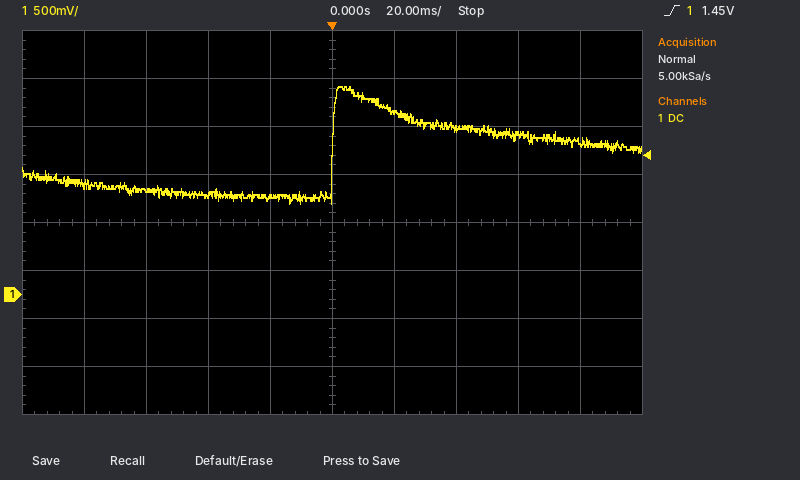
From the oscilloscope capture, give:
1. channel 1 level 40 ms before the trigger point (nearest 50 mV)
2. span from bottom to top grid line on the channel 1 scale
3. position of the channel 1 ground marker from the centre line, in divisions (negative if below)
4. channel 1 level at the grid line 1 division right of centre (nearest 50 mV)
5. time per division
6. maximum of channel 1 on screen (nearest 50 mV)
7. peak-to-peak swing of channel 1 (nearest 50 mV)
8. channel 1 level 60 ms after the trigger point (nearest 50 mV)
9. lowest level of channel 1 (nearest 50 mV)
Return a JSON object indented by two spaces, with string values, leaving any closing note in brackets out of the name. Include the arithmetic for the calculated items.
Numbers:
{
  "channel 1 level 40 ms before the trigger point": "1.05 V",
  "span from bottom to top grid line on the channel 1 scale": "4 V",
  "position of the channel 1 ground marker from the centre line, in divisions": "-1.5 div",
  "channel 1 level at the grid line 1 division right of centre": "1.90 V",
  "time per division": "20 ms",
  "maximum of channel 1 on screen": "2.15 V",
  "peak-to-peak swing of channel 1": "2.15 V − (950 mV) = 1.20 V",
  "channel 1 level 60 ms after the trigger point": "1.65 V",
  "lowest level of channel 1": "950 mV"
}
